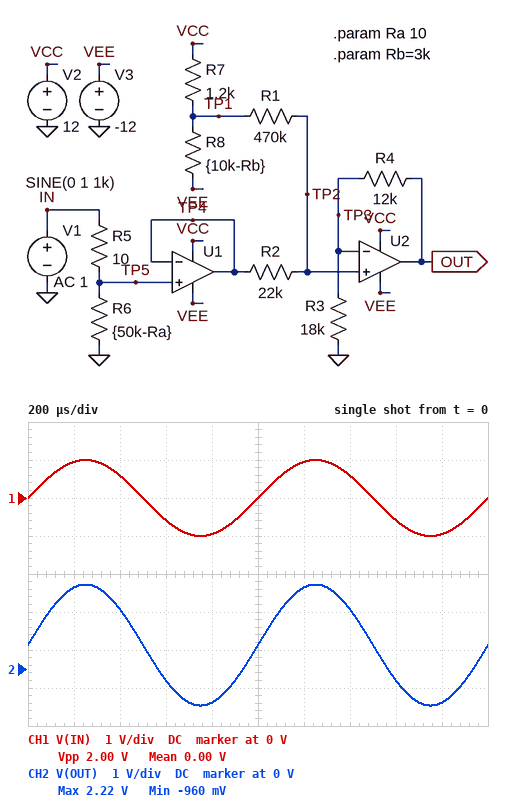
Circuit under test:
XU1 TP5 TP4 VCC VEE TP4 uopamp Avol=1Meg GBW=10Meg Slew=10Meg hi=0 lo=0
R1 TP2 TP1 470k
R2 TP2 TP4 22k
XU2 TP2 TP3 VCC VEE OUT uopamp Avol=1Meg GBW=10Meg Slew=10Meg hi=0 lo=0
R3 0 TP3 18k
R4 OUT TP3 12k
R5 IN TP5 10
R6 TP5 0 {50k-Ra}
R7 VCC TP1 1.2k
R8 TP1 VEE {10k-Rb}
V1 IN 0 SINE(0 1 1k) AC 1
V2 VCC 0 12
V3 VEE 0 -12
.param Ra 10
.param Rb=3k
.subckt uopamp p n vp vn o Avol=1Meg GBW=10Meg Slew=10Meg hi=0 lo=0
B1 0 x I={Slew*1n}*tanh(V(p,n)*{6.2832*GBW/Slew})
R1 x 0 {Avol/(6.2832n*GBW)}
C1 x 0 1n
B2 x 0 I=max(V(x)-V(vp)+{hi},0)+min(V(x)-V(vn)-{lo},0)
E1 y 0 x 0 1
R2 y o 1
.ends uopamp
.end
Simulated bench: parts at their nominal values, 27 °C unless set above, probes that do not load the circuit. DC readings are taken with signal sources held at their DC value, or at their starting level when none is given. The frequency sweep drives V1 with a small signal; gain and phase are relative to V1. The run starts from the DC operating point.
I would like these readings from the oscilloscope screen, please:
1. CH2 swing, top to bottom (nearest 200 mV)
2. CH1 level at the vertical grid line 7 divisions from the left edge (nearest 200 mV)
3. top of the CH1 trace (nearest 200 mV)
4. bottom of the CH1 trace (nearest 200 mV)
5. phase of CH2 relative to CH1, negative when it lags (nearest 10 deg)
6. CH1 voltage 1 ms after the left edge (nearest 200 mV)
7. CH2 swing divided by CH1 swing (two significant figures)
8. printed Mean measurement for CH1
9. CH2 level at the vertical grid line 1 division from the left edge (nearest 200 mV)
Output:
3.2 V
600 mV
1.0 V
-1.0 V
0 deg
0 V
1.6
0.00 V
2.2 V
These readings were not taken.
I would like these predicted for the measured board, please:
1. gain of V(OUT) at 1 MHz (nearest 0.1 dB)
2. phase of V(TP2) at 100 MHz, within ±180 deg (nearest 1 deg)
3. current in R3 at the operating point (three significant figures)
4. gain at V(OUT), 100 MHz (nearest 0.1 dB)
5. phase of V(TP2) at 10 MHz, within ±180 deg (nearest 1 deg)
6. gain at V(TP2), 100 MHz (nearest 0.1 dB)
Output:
3.9 dB
-84 deg
21.0 µA
-40.5 dB
-45 deg
-20.4 dB
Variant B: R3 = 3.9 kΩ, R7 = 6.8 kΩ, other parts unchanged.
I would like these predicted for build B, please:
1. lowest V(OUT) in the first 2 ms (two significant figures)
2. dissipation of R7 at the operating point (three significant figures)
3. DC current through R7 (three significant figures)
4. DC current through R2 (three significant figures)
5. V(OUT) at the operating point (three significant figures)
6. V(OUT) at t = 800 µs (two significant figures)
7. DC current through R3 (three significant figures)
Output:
-3.9 V
20.6 mW
1.74 mA
351 nA
31.5 mV
-3.7 V
1.98 µA
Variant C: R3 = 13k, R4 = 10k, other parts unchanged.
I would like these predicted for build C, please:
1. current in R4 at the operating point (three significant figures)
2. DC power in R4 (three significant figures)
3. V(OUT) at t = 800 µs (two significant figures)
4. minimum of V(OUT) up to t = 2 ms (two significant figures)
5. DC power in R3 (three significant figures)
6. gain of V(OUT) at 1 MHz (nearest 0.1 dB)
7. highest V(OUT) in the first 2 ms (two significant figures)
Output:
29.1 µA
8.49 µW
-940 mV
-1.0 V
11.0 µW
4.4 dB
2.4 V
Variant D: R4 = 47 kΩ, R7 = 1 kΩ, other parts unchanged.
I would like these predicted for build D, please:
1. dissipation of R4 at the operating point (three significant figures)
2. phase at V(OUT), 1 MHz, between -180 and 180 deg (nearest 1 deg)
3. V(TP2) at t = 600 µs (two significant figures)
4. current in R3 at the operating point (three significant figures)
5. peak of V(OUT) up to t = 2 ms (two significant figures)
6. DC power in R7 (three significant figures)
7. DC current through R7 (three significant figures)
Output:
23.4 µW
-26 deg
-160 mV
22.3 µA
4.9 V
9.10 mW
3.02 mA
